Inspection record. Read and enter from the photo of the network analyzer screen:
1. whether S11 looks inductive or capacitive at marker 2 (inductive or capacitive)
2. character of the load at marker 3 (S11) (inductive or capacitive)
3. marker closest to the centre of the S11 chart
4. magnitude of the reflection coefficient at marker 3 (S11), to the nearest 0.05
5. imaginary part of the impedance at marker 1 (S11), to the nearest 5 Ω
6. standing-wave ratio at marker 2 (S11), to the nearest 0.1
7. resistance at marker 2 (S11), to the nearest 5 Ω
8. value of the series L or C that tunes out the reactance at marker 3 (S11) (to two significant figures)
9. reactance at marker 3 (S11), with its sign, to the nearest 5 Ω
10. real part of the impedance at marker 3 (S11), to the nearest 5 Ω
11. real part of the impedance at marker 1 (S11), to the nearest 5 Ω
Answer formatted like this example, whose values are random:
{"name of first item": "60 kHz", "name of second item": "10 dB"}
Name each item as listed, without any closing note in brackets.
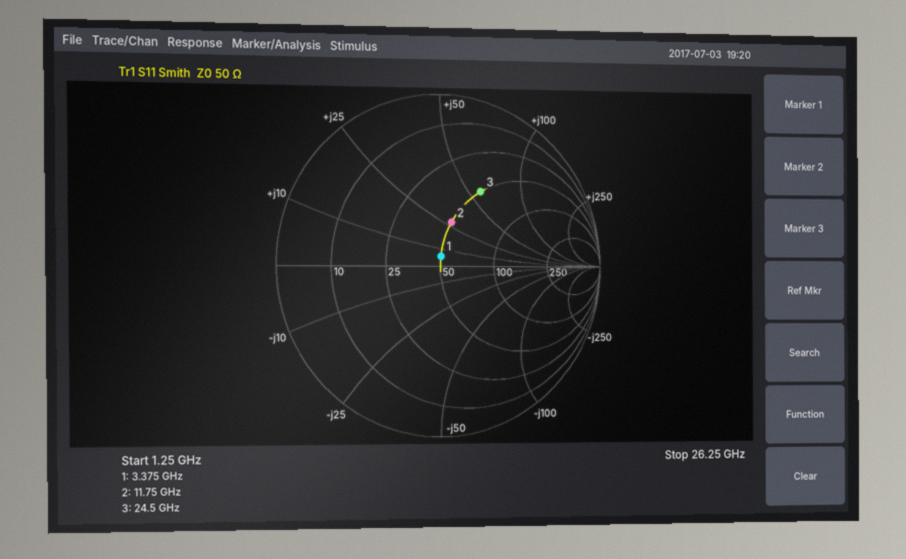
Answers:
{"whether S11 looks inductive or capacitive at marker 2": "inductive", "character of the load at marker 3 (S11)": "inductive", "marker closest to the centre of the S11 chart": "marker 1", "magnitude of the reflection coefficient at marker 3 (S11), to the nearest 0.05": "0.50", "imaginary part of the impedance at marker 1 (S11), to the nearest 5 Ω": "+5 Ω", "standing-wave ratio at marker 2 (S11), to the nearest 0.1": "1.7", "resistance at marker 2 (S11), to the nearest 5 Ω": "50 Ω", "value of the series L or C that tunes out the reactance at marker 3 (S11)": "110 fF", "reactance at marker 3 (S11), with its sign, to the nearest 5 Ω": "+60 Ω", "real part of the impedance at marker 3 (S11), to the nearest 5 Ω": "50 Ω", "real part of the impedance at marker 1 (S11), to the nearest 5 Ω": "50 Ω"}
